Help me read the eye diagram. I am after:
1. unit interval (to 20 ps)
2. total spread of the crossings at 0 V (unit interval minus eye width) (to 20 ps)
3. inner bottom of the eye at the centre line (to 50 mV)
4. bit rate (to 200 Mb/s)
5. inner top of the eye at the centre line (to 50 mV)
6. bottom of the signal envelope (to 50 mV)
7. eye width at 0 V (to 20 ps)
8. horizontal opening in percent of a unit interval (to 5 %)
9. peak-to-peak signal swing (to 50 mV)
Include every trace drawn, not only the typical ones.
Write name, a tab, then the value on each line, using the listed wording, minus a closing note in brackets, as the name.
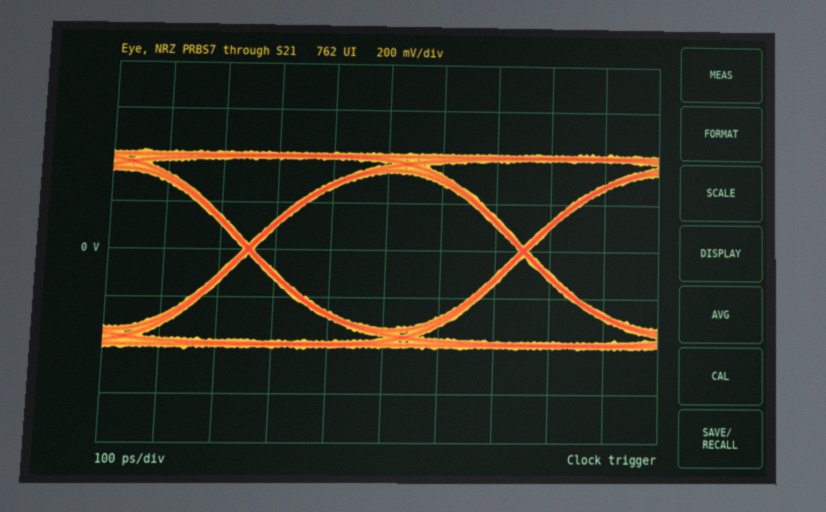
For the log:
unit interval	500 ps
total spread of the crossings at 0 V (unit interval minus eye width)	20 ps
inner bottom of the eye at the centre line	-350 mV
bit rate	2.0 Gb/s
inner top of the eye at the centre line	350 mV
bottom of the signal envelope	-400 mV
eye width at 0 V	480 ps
horizontal opening in percent of a unit interval	95 %
peak-to-peak signal swing	850 mV
